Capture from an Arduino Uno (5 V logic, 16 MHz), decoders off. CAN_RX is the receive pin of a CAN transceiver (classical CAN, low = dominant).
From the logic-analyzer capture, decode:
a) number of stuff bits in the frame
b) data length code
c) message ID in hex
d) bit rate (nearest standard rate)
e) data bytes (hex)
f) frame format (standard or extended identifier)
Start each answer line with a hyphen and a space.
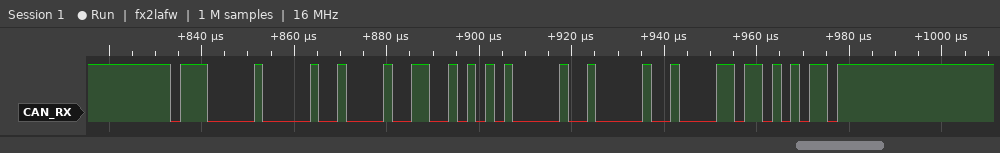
- 4
- 4
- 0x700
- 500 kbit/s
- 26 55 01 01
- standard
